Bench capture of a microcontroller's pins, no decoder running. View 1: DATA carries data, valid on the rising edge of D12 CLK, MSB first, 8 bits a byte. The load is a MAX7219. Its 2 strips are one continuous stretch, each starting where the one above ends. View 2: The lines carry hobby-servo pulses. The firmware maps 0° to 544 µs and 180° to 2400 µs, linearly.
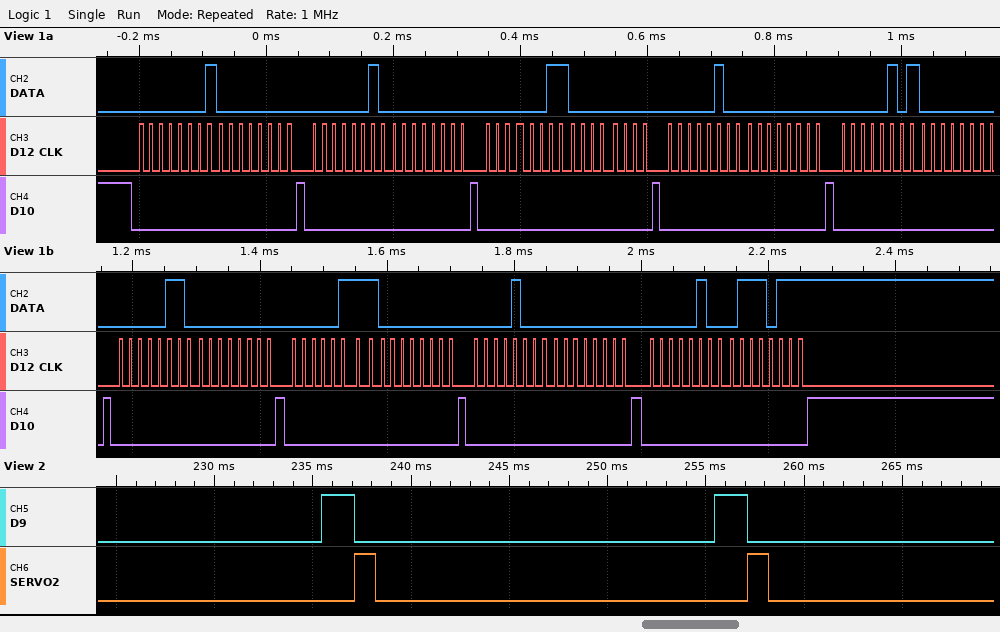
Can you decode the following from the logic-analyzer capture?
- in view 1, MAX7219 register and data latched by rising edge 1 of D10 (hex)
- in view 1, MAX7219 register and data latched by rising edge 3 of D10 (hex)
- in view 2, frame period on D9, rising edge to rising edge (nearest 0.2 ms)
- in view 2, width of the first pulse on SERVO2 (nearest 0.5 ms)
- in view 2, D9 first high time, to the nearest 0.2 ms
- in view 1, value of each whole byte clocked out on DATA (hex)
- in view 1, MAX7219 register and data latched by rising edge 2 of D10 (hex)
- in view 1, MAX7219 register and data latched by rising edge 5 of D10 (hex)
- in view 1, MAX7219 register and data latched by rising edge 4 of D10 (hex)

register 0x1, data 0x00
register 0x3, data 0x00
20.0 ms
1.0 ms
1.6 ms
01 00 02 00 03 00 04 00 05 00 06 00 07 00 08 00 04 77
register 0x2, data 0x00
register 0x5, data 0x00
register 0x4, data 0x00
